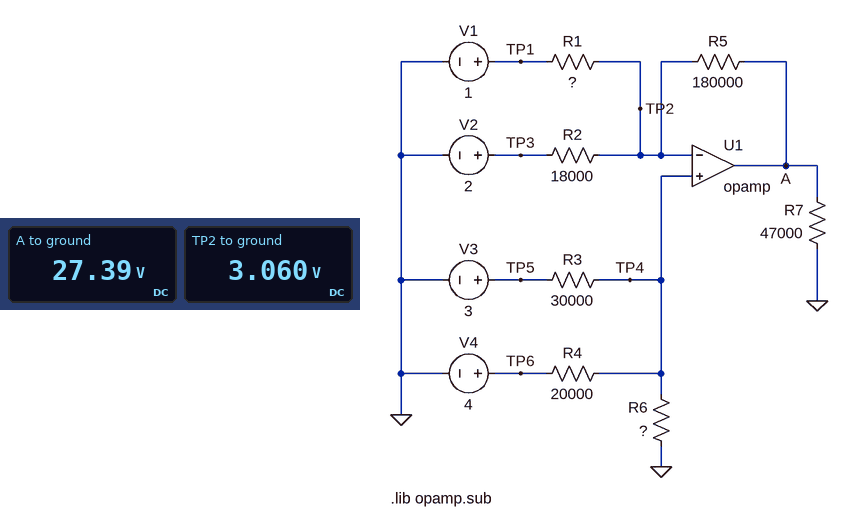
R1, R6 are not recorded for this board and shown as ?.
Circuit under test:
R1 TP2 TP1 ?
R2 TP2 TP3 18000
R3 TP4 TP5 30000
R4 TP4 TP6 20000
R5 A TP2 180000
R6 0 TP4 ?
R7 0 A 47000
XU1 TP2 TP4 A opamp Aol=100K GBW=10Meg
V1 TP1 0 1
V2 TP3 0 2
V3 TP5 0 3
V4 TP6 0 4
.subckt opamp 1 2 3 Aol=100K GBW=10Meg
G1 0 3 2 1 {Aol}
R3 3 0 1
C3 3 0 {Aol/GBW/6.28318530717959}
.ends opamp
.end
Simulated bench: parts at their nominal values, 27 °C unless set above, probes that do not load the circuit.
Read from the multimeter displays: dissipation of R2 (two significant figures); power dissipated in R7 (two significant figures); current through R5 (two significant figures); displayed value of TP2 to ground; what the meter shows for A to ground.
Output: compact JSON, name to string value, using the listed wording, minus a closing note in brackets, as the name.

{"dissipation of R2": "62 µW", "power dissipated in R7": "16 mW", "current through R5": "140 µA", "displayed value of TP2 to ground": "3.060 V", "what the meter shows for A to ground": "27.39 V"}
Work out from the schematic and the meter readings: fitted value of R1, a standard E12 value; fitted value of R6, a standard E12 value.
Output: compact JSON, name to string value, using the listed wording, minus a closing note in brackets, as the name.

{"fitted value of R1, a standard E12 value": "27 kΩ", "fitted value of R6, a standard E12 value": "68 kΩ"}
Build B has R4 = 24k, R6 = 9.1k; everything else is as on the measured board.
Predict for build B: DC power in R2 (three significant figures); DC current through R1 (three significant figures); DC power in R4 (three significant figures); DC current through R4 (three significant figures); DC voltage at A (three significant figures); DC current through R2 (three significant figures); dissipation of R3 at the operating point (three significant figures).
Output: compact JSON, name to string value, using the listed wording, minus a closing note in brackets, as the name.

{"DC power in R2": "17.3 µW", "DC current through R1": "16.4 µA", "DC power in R4": "273 µW", "DC current through R4": "107 µA", "DC voltage at A": "-1.19 V", "DC current through R2": "31.0 µA", "dissipation of R3 at the operating point": "80.9 µW"}
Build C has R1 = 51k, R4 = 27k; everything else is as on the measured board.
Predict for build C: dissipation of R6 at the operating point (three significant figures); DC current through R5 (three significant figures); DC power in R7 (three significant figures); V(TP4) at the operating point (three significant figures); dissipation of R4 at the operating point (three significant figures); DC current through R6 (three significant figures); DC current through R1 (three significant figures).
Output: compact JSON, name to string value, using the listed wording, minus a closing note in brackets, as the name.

{"dissipation of R6 at the operating point": "125 µW", "DC current through R5": "88.5 µA", "DC power in R7": "7.56 mW", "V(TP4) at the operating point": "2.92 V", "dissipation of R4 at the operating point": "43.5 µW", "DC current through R6": "42.9 µA", "DC current through R1": "37.6 µA"}
